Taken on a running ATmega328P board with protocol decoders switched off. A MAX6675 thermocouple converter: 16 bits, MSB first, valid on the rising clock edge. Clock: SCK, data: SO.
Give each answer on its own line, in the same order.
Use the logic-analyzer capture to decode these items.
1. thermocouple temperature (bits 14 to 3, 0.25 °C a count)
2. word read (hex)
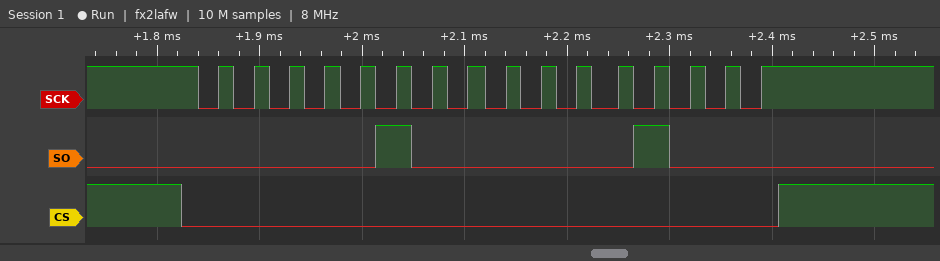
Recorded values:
32.25 °C
0x0408
